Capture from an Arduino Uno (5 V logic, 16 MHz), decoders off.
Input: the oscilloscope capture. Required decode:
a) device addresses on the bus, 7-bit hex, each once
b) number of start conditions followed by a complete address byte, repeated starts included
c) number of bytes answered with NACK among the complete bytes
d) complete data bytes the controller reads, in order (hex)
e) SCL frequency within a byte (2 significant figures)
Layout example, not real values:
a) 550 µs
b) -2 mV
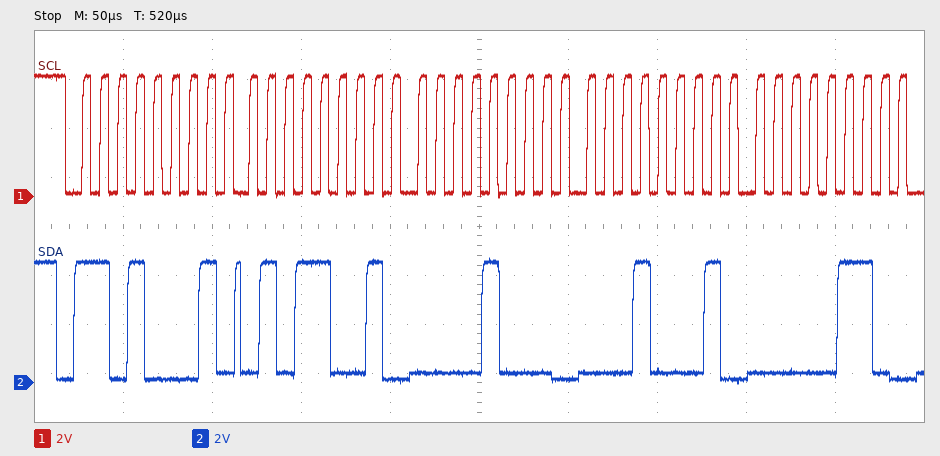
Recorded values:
a) 0x68
b) 1
c) 0
d) 59 08 11 06
e) 100 kHz
